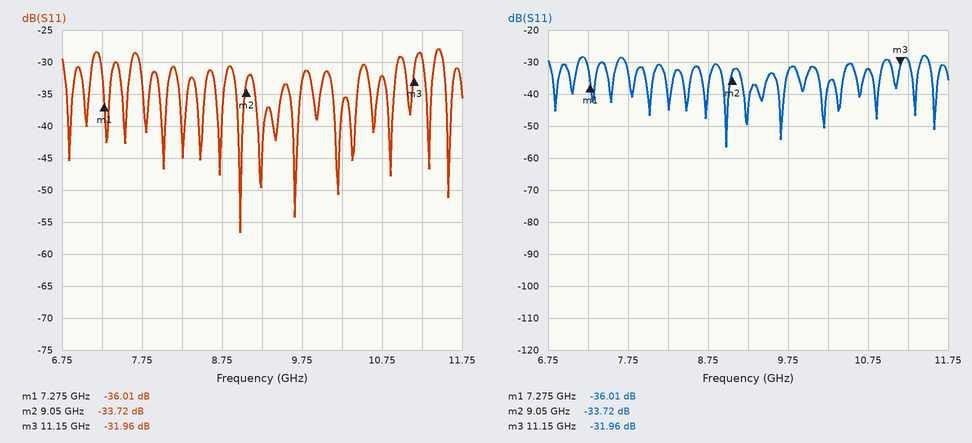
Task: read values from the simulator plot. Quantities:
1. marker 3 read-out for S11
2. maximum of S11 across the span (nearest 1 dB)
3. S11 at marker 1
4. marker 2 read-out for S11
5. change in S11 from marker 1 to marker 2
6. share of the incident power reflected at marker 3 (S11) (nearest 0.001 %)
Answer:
-31.96 dB
-28 dB
-36.01 dB
-33.72 dB
2.29 dB
0.064 %
